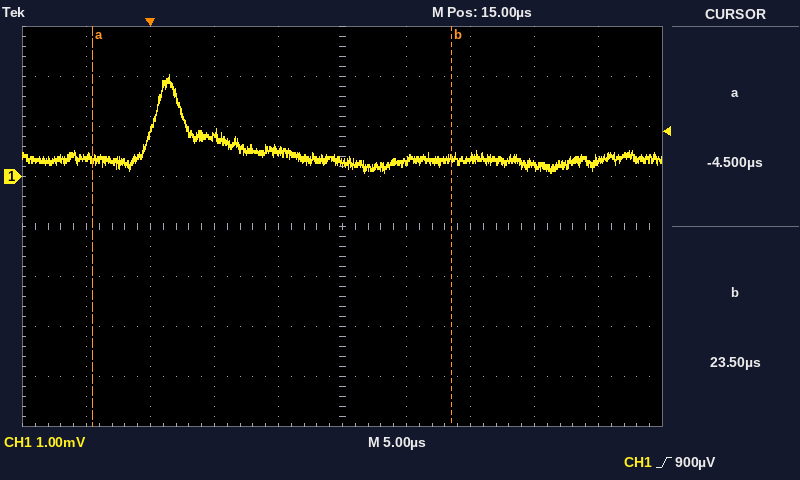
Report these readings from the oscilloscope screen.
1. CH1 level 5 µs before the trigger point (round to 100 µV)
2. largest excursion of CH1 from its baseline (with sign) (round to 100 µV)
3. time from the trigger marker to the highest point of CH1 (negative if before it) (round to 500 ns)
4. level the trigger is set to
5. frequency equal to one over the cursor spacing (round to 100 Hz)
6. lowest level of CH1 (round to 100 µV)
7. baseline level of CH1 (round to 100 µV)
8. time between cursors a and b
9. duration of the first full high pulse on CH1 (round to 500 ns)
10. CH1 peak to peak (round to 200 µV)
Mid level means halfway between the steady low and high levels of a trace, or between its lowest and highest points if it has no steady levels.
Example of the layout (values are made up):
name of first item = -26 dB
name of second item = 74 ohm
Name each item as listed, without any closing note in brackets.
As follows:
CH1 level 5 µs before the trigger point = 400 µV
largest excursion of CH1 from its baseline (with sign) = +1.7 mV
time from the trigger marker to the highest point of CH1 (negative if before it) = +1.5 µs
level the trigger is set to = 900 µV
frequency equal to one over the cursor spacing = 35.7 kHz
lowest level of CH1 = 100 µV
baseline level of CH1 = 300 µV
time between cursors a and b = 28.0 µs
duration of the first full high pulse on CH1 = 2.5 µs
CH1 peak to peak = 2.0 mV
